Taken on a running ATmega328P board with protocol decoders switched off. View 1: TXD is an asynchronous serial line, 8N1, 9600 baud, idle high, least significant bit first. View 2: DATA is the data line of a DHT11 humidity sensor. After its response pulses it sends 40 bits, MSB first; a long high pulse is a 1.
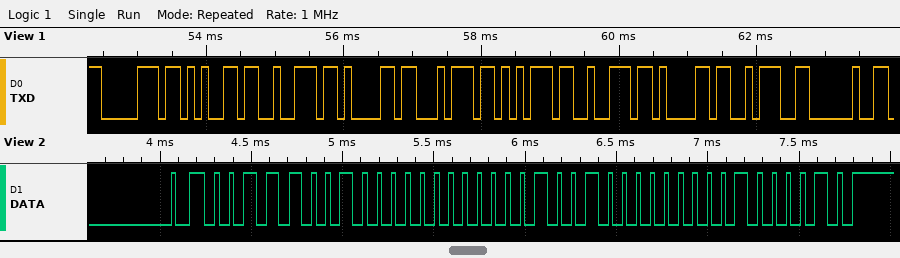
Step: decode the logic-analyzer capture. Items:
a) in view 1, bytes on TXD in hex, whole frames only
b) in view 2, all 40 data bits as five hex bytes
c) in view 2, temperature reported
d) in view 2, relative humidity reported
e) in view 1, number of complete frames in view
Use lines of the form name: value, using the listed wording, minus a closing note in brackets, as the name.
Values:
in view 1, bytes on TXD in hex, whole frames only: 70 65 72 61 74 75 72 61 3A 20
in view 2, all 40 data bits as five hex bytes: 39 00 09 00 42
in view 2, temperature reported: 9.0 °C
in view 2, relative humidity reported: 57 %
in view 1, number of complete frames in view: 10
